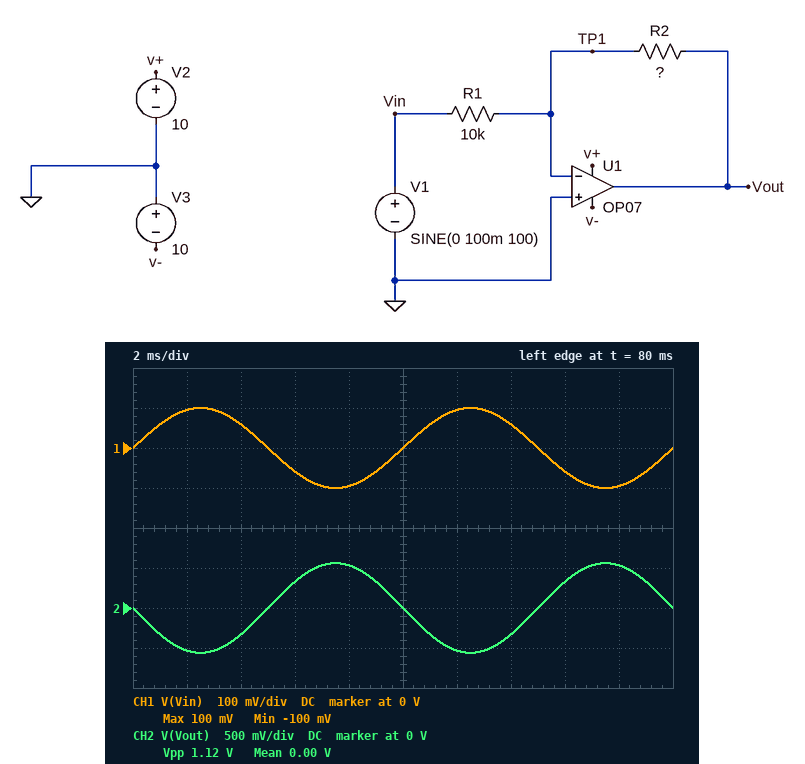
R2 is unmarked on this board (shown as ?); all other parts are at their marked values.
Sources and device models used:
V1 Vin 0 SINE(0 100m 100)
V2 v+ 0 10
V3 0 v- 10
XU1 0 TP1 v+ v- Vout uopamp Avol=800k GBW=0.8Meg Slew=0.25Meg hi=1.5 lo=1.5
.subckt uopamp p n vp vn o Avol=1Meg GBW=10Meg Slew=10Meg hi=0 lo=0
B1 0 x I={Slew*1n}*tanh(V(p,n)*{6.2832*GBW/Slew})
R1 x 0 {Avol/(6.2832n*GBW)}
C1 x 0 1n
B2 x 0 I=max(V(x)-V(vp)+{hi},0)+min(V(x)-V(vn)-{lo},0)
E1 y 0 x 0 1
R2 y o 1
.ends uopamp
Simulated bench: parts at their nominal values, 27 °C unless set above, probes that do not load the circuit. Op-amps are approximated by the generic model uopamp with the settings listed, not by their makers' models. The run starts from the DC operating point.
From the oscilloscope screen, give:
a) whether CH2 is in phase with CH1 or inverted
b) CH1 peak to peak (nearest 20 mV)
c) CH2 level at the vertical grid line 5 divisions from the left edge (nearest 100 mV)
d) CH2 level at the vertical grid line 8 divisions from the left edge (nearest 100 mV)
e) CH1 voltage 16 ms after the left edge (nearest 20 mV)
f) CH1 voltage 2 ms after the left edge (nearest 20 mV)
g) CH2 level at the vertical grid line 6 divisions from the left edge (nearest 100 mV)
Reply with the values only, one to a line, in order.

inverted
200 mV
0 V
300 mV
-60 mV
100 mV
-500 mV
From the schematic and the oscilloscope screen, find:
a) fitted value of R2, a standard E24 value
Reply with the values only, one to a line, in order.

56 kΩ
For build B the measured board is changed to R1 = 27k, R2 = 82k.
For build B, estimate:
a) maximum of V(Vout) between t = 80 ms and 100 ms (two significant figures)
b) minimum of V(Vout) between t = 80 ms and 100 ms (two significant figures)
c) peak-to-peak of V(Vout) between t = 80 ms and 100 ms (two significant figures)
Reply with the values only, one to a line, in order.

300 mV
-300 mV
610 mV
